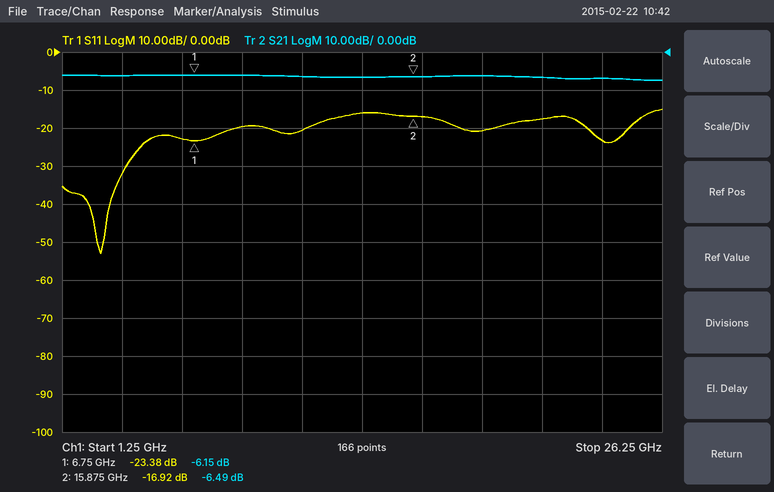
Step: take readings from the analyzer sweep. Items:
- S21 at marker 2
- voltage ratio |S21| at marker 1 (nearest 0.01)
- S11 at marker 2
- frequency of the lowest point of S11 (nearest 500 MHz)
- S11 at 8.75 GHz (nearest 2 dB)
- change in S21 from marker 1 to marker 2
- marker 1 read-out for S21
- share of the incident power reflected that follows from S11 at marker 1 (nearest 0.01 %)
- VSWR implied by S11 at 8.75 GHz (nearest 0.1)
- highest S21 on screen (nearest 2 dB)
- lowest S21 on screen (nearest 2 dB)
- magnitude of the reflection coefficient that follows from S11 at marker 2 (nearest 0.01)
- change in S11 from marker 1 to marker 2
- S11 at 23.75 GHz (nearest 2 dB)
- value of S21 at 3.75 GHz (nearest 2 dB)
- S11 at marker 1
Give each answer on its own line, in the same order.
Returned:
-6.49 dB
0.49
-16.92 dB
3.0 GHz
-20 dB
-0.34 dB
-6.15 dB
0.46 %
1.2
-6 dB
-8 dB
0.14
6.46 dB
-24 dB
-6 dB
-23.38 dB
